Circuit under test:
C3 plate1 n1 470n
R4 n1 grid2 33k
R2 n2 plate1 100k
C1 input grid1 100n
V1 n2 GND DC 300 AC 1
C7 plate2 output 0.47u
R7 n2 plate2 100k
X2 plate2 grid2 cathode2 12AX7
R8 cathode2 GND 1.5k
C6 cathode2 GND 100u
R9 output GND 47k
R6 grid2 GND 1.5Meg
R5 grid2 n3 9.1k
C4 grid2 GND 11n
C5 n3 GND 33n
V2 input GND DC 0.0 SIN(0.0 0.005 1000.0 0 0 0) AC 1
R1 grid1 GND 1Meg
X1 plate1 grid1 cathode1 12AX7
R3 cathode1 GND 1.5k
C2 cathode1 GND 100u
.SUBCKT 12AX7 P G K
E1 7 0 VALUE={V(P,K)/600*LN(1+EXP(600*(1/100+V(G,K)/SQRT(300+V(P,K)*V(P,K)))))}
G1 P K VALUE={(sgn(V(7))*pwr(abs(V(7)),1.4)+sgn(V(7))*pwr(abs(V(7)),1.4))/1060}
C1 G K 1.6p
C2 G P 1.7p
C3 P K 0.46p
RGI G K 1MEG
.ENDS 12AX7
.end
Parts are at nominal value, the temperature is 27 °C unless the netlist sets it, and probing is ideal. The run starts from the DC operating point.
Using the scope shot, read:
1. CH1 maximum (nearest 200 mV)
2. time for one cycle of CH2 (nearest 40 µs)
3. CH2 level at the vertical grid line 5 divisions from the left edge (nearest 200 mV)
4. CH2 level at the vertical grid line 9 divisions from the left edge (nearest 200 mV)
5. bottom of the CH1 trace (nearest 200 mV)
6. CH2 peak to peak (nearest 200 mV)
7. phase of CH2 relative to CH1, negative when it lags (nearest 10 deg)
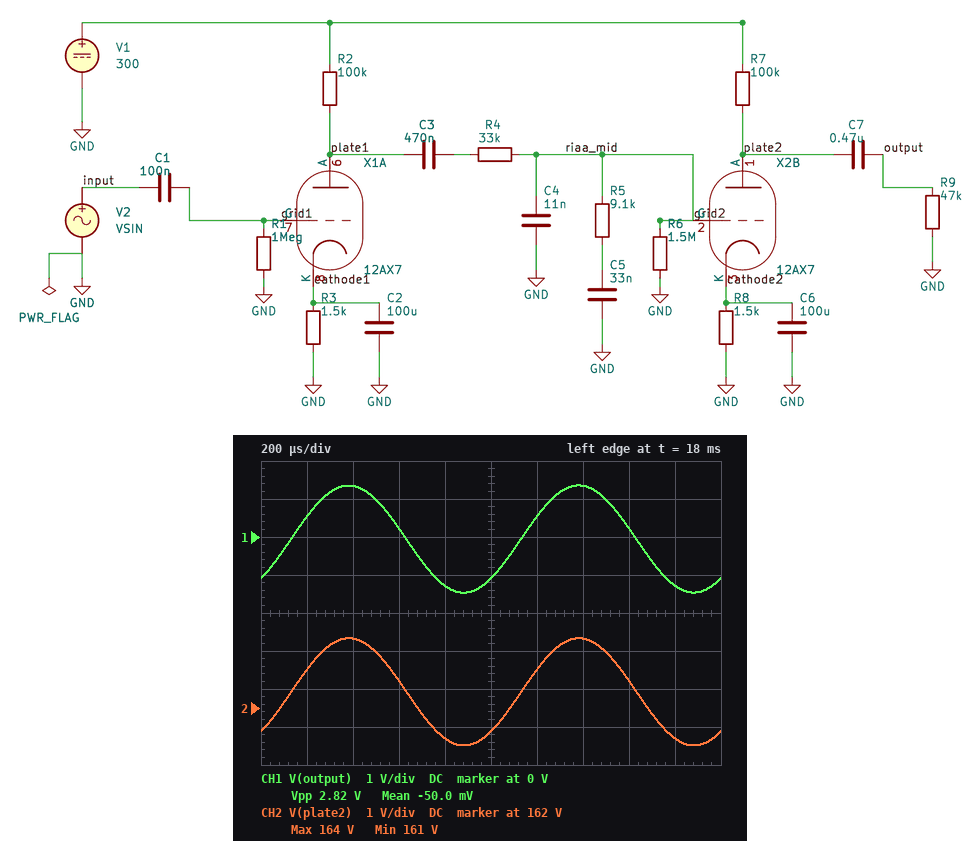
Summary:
1.4 V
1.00 ms
161.4 V
161.2 V
-1.4 V
2.8 V
0 deg
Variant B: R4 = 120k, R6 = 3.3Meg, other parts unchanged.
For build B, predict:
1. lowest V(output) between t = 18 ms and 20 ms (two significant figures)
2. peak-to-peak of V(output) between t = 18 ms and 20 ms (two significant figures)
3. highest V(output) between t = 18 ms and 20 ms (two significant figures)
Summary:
-690 mV
1.3 V
600 mV
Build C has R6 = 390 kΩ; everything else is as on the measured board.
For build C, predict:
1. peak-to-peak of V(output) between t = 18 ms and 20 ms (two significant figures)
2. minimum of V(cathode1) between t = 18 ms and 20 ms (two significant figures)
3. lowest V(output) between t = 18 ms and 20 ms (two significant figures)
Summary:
2.6 V
1.9 V
-1.3 V
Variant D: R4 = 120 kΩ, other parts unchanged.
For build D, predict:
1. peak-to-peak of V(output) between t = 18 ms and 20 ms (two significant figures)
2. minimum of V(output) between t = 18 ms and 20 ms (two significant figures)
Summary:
1.2 V
-660 mV
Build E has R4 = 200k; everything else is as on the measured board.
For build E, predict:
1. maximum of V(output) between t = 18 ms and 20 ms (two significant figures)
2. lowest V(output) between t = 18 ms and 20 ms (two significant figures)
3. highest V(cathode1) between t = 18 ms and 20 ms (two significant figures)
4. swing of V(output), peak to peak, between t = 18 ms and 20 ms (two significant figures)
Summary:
370 mV
-440 mV
1.9 V
820 mV
